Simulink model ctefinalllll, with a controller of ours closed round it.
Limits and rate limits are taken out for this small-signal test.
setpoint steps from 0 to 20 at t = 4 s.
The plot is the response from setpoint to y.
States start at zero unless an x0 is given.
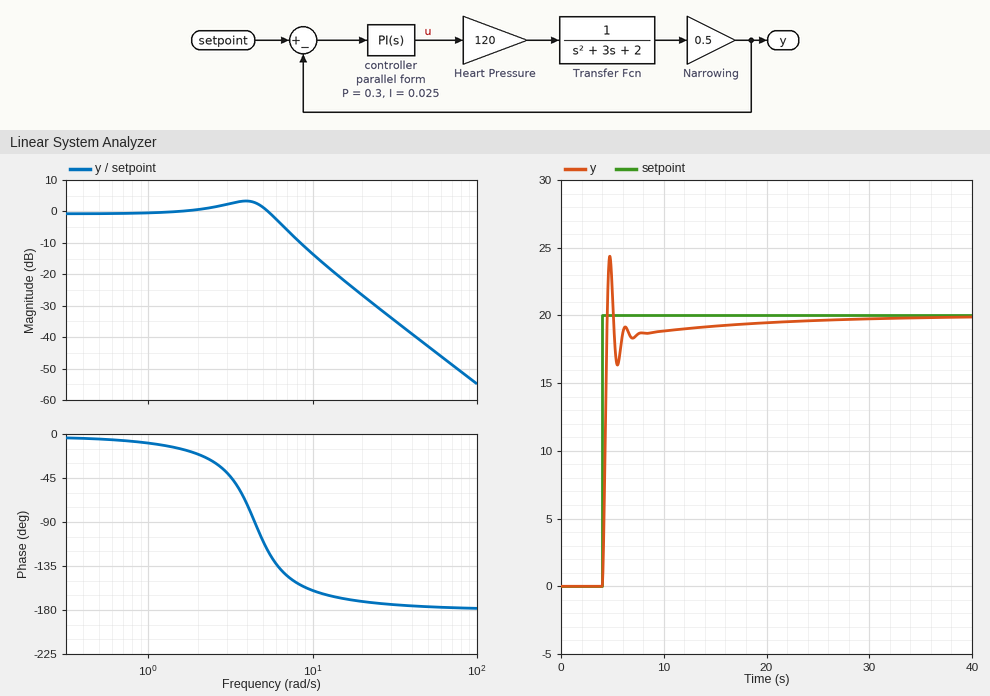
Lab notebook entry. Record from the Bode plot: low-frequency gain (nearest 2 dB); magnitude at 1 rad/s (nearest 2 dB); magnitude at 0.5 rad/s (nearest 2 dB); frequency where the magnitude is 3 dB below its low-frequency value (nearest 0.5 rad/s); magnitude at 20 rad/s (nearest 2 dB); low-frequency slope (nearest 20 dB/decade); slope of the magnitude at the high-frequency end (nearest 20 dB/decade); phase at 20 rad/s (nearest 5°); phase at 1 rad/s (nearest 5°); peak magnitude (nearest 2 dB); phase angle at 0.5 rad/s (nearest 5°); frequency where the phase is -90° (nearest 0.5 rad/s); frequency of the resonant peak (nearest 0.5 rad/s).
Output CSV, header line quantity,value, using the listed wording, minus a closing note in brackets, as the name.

quantity,value
low-frequency gain,0 dB
magnitude at 1 rad/s,0 dB
magnitude at 0.5 rad/s,0 dB
frequency where the magnitude is 3 dB below its low-frequency value,6.5 rad/s
magnitude at 20 rad/s,-26 dB
low-frequency slope,0 dB/decade
slope of the magnitude at the high-frequency end,-40 dB/decade
phase at 20 rad/s,-170°
phase at 1 rad/s,-10°
peak magnitude,4 dB
phase angle at 0.5 rad/s,-5°
frequency where the phase is -90°,4.5 rad/s
frequency of the resonant peak,4.0 rad/s
